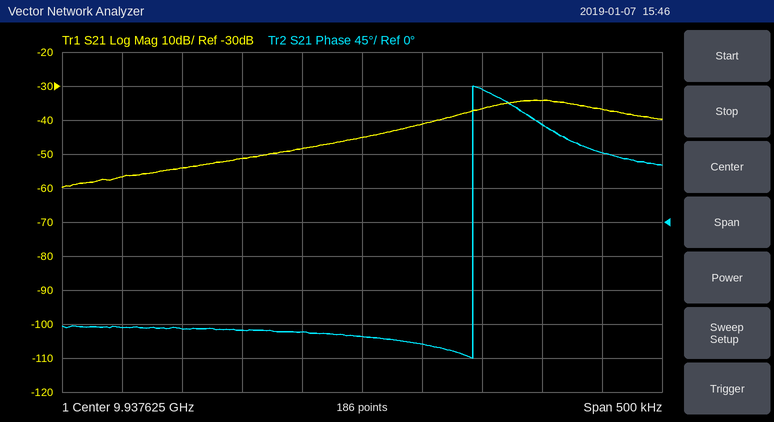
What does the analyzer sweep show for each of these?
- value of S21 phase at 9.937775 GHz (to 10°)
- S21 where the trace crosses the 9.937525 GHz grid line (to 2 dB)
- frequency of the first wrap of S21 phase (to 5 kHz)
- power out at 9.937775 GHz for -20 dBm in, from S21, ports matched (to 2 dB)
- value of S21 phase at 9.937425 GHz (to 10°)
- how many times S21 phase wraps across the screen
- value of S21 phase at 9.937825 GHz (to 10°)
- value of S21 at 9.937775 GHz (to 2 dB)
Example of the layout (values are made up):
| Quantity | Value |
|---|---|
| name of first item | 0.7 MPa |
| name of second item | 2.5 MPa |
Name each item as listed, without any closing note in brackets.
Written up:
| Quantity | Value |
|---|---|
| value of S21 phase at 9.937775 GHz | 130° |
| S21 where the trace crosses the 9.937525 GHz grid line | -52 dB |
| frequency of the first wrap of S21 phase | 9.937715 GHz |
| power out at 9.937775 GHz for -20 dBm in, from S21, ports matched | -54 dBm |
| value of S21 phase at 9.937425 GHz | -140° |
| how many times S21 phase wraps across the screen | 1 |
| value of S21 phase at 9.937825 GHz | 90° |
| value of S21 at 9.937775 GHz | -34 dB |
